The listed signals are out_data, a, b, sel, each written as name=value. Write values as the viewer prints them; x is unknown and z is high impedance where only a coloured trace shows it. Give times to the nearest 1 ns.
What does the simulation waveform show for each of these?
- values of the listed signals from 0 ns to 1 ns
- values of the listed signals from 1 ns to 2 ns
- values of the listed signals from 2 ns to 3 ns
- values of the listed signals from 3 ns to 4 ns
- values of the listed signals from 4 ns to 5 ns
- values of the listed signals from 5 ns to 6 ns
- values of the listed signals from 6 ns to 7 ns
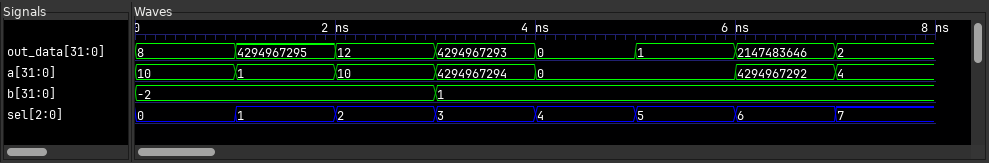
out_data=8, a=10, b=-2, sel=0
out_data=4294967295, a=1, b=-2, sel=1
out_data=12, a=10, b=-2, sel=2
out_data=4294967293, a=4294967294, b=1, sel=3
out_data=0, a=0, b=1, sel=4
out_data=1, a=0, b=1, sel=5
out_data=2147483646, a=4294967292, b=1, sel=6
